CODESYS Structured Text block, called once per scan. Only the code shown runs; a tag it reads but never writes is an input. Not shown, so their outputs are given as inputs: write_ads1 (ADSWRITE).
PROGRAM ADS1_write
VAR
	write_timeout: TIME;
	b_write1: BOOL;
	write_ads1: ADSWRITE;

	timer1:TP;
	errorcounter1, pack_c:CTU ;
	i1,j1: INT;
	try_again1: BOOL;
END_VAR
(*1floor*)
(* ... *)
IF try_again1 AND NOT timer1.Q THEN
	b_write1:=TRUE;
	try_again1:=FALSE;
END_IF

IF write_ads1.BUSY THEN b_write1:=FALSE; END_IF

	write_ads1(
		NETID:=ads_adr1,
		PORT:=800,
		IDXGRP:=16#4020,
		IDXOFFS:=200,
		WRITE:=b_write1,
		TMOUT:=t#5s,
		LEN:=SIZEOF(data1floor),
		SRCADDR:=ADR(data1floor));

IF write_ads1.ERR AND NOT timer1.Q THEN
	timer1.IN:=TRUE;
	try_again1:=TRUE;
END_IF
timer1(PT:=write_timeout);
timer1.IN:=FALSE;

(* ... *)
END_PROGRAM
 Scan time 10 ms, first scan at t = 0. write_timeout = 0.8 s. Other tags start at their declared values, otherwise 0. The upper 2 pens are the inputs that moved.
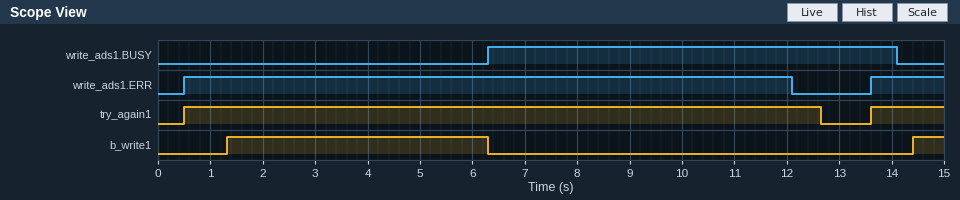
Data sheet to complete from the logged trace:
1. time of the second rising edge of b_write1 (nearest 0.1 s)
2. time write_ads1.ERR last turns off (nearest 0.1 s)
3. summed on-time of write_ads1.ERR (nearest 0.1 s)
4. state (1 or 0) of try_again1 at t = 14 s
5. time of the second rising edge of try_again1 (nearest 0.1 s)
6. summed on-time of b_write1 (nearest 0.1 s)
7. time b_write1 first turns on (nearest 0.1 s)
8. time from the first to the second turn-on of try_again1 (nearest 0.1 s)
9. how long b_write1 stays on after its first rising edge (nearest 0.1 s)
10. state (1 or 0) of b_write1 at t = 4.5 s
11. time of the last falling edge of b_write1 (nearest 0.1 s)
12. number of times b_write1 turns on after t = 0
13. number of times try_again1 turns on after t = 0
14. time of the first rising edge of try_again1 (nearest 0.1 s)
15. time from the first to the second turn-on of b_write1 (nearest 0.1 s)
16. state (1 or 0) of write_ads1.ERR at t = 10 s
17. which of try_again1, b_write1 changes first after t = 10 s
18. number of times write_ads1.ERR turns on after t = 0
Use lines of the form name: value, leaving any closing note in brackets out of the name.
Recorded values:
time of the second rising edge of b_write1: 14.4 s
time write_ads1.ERR last turns off: 12.1 s
summed on-time of write_ads1.ERR: 13.0 s
state (1 or 0) of try_again1 at t = 14 s: 1
time of the second rising edge of try_again1: 13.6 s
summed on-time of b_write1: 5.6 s
time b_write1 first turns on: 1.3 s
time from the first to the second turn-on of try_again1: 13.1 s
how long b_write1 stays on after its first rising edge: 5.0 s
state (1 or 0) of b_write1 at t = 4.5 s: 1
time of the last falling edge of b_write1: 6.3 s
number of times b_write1 turns on after t = 0: 2
number of times try_again1 turns on after t = 0: 2
time of the first rising edge of try_again1: 0.5 s
time from the first to the second turn-on of b_write1: 13.1 s
state (1 or 0) of write_ads1.ERR at t = 10 s: 1
which of try_again1, b_write1 changes first after t = 10 s: try_again1
number of times write_ads1.ERR turns on after t = 0: 2
